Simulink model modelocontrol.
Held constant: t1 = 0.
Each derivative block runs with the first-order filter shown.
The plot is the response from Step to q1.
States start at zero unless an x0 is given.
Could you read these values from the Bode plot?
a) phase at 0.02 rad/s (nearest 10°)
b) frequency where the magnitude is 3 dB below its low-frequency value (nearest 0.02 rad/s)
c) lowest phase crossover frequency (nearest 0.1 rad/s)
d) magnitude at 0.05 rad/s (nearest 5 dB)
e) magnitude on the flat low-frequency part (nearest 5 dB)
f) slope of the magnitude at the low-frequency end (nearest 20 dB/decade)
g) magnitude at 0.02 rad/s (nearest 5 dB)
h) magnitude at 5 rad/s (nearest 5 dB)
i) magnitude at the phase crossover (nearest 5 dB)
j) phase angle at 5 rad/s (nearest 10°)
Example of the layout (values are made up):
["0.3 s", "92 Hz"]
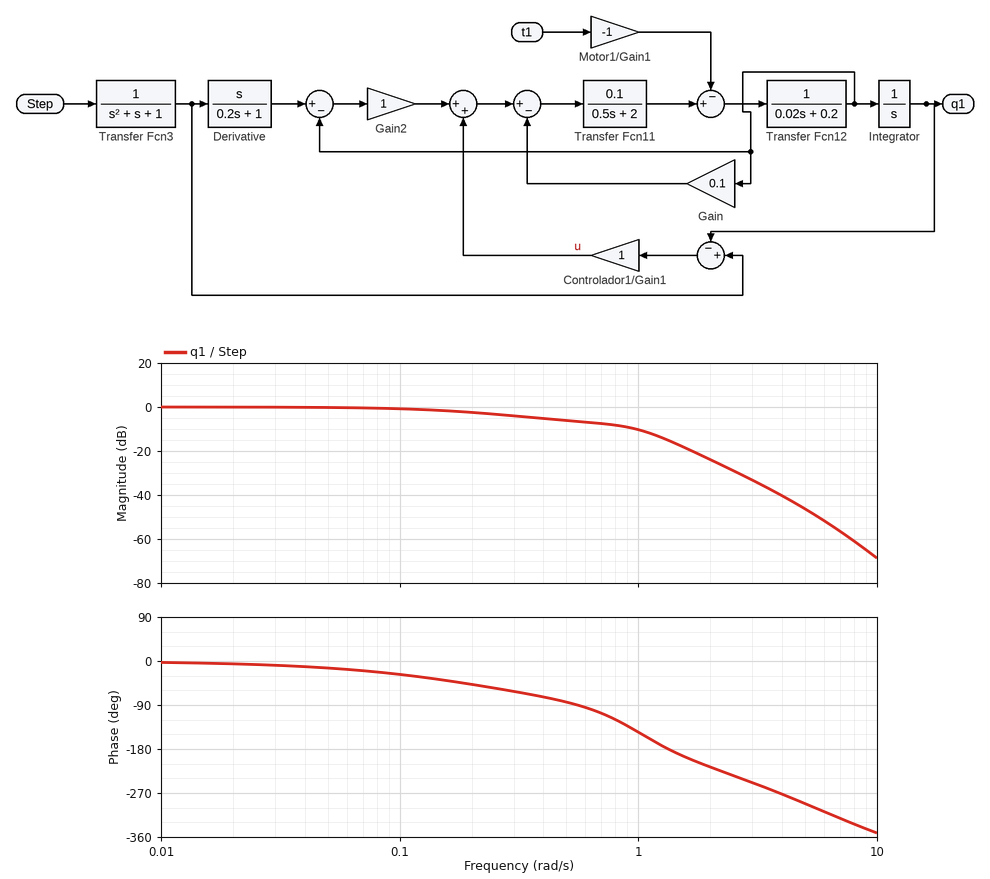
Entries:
["-10°", "0.24 rad/s", "1.3 rad/s", "0 dB", "0 dB", "0 dB/decade", "0 dB", "-45 dB", "-15 dB", "-290°"]
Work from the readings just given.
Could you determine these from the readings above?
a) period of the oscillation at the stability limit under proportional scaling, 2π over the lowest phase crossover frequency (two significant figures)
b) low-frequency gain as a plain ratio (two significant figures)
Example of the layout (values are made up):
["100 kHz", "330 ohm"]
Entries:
["4.8 s", "1.0"]
